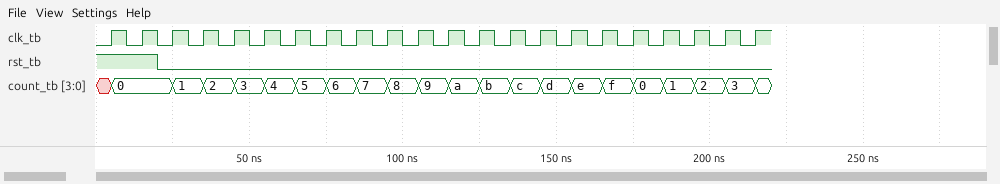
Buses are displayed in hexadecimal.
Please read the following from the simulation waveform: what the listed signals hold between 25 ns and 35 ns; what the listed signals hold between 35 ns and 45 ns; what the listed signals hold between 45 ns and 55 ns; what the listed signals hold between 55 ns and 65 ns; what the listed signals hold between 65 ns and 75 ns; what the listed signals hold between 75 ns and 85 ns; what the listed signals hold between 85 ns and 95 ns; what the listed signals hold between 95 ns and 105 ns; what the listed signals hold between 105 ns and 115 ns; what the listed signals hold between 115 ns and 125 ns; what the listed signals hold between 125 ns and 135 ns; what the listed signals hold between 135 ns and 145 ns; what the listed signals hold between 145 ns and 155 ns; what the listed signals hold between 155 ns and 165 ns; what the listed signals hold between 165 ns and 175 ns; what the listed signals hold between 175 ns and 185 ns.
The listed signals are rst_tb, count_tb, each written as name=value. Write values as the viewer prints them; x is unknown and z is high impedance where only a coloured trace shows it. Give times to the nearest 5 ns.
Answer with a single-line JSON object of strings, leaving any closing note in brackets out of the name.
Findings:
{"what the listed signals hold between 25 ns and 35 ns": "rst_tb=0, count_tb=1", "what the listed signals hold between 35 ns and 45 ns": "rst_tb=0, count_tb=2", "what the listed signals hold between 45 ns and 55 ns": "rst_tb=0, count_tb=3", "what the listed signals hold between 55 ns and 65 ns": "rst_tb=0, count_tb=4", "what the listed signals hold between 65 ns and 75 ns": "rst_tb=0, count_tb=5", "what the listed signals hold between 75 ns and 85 ns": "rst_tb=0, count_tb=6", "what the listed signals hold between 85 ns and 95 ns": "rst_tb=0, count_tb=7", "what the listed signals hold between 95 ns and 105 ns": "rst_tb=0, count_tb=8", "what the listed signals hold between 105 ns and 115 ns": "rst_tb=0, count_tb=9", "what the listed signals hold between 115 ns and 125 ns": "rst_tb=0, count_tb=a", "what the listed signals hold between 125 ns and 135 ns": "rst_tb=0, count_tb=b", "what the listed signals hold between 135 ns and 145 ns": "rst_tb=0, count_tb=c", "what the listed signals hold between 145 ns and 155 ns": "rst_tb=0, count_tb=d", "what the listed signals hold between 155 ns and 165 ns": "rst_tb=0, count_tb=e", "what the listed signals hold between 165 ns and 175 ns": "rst_tb=0, count_tb=f", "what the listed signals hold between 175 ns and 185 ns": "rst_tb=0, count_tb=0"}
